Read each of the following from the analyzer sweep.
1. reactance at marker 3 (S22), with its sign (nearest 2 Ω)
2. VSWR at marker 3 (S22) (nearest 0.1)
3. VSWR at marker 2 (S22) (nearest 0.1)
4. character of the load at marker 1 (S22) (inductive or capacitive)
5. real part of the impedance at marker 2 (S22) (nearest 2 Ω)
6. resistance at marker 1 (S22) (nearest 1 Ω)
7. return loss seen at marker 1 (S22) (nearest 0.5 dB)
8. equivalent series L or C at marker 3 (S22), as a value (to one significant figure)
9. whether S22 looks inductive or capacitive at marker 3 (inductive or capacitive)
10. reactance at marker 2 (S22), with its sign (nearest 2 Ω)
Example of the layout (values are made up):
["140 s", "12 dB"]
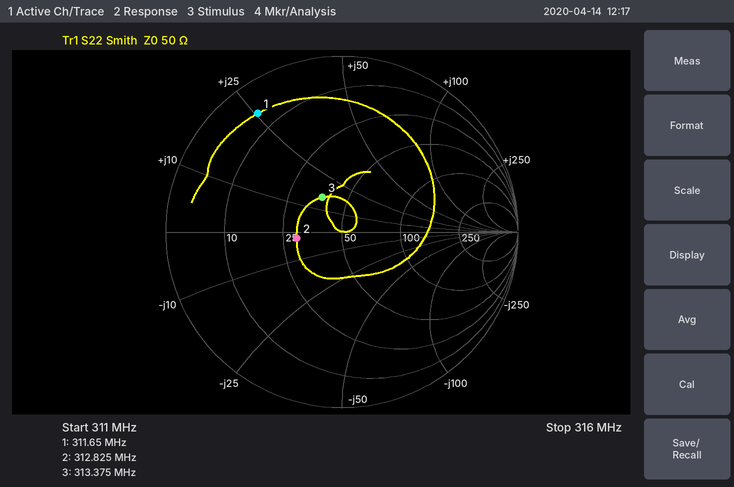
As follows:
["+16 Ω", "1.6", "1.7", "inductive", "30 Ω", "6 Ω", "1.5 dB", "8 nH", "inductive", "-2 Ω"]
